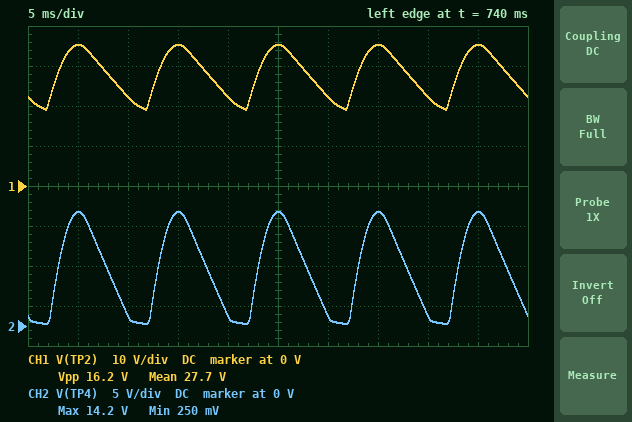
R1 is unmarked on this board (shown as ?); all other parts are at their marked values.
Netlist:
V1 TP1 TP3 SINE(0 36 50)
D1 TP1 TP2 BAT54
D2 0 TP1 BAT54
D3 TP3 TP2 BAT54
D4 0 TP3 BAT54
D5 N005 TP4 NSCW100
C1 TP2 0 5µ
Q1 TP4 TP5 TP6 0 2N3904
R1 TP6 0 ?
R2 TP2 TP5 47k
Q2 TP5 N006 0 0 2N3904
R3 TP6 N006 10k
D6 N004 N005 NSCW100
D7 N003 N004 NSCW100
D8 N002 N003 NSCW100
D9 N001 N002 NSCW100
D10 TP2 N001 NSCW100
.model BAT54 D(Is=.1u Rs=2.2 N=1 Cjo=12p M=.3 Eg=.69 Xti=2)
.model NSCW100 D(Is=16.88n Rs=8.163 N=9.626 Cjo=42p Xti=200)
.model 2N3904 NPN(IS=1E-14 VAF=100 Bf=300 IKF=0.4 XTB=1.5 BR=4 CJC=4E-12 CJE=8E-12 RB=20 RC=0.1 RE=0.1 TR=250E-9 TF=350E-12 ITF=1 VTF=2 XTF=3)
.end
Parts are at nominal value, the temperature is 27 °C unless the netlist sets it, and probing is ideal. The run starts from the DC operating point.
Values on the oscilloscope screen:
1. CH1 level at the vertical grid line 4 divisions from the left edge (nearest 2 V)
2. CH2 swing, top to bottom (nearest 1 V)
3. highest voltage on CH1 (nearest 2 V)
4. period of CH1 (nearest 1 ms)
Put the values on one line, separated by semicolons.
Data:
22 V; 14 V; 36 V; 10 ms
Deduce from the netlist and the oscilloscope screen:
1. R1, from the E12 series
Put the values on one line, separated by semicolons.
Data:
47 Ω
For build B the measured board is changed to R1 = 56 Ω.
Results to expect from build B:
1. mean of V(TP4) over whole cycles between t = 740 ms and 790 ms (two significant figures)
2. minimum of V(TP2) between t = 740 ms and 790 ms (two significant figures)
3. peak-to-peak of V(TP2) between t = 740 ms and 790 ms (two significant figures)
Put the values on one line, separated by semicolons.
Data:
7.8 V; 20 V; 15 V
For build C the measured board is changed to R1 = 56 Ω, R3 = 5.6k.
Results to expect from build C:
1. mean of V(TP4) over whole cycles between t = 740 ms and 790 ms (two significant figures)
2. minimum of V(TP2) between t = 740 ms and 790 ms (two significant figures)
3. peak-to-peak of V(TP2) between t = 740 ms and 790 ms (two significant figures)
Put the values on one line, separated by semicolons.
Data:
7.9 V; 20 V; 15 V
